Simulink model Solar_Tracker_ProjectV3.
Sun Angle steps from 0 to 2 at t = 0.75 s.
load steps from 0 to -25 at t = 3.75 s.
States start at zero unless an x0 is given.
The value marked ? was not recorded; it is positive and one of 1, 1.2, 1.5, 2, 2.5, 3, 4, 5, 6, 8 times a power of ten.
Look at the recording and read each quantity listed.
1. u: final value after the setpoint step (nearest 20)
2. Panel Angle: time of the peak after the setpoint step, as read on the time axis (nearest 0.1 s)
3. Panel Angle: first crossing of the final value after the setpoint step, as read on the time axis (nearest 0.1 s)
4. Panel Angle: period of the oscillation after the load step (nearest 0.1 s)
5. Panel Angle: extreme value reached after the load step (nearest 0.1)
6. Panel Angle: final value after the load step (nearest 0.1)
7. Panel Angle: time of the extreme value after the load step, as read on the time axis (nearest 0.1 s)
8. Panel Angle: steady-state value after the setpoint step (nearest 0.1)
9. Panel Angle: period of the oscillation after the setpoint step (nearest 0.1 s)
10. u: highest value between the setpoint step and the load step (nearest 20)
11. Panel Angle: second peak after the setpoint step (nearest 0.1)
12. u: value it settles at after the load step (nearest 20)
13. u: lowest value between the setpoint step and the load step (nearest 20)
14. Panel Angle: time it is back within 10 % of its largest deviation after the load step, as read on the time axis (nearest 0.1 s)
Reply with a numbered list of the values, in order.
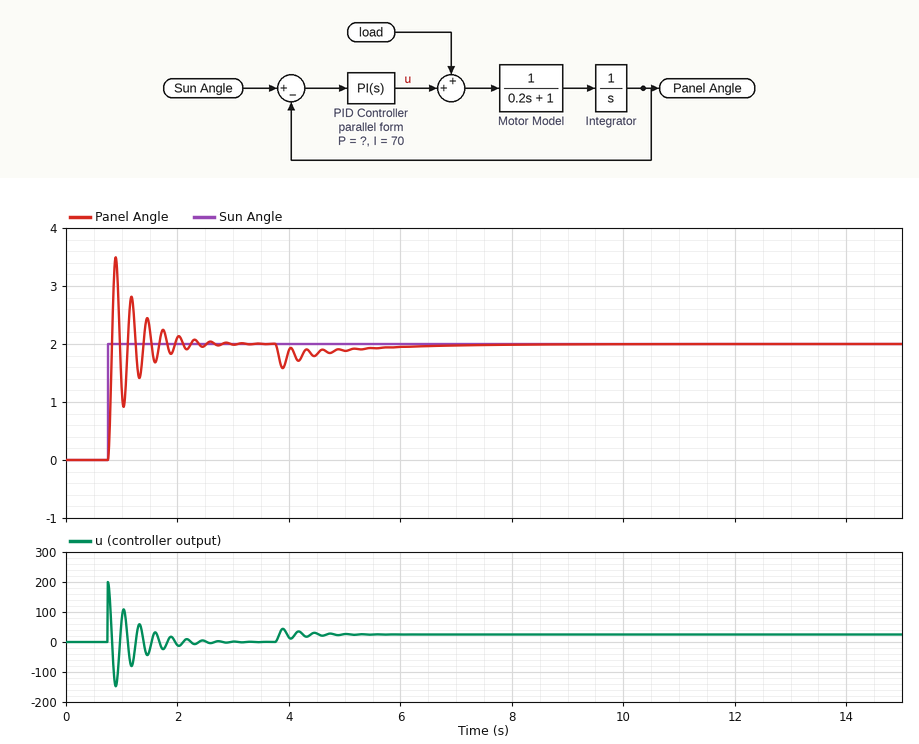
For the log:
1. 0
2. 0.9 s
3. 0.8 s
4. 0.3 s
5. 1.6
6. 2.0
7. 3.9 s
8. 2.0
9. 0.3 s
10. 200
11. 2.8
12. 20
13. -140
14. 6.3 s
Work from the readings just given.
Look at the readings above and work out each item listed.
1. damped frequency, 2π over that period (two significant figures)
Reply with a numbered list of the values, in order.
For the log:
1. 21 rad/s
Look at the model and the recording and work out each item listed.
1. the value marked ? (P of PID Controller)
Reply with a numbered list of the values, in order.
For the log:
1. 100
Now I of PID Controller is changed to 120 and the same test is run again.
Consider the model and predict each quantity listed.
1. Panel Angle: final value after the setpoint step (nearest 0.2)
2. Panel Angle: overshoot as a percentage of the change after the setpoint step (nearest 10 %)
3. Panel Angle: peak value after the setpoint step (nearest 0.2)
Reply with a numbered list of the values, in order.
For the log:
1. 2.0
2. 80 %
3. 3.6
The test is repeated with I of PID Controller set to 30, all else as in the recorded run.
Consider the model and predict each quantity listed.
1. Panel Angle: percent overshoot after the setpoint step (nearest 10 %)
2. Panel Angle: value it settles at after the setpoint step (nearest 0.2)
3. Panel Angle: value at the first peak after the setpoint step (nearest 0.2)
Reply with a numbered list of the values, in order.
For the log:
1. 70 %
2. 2.0
3. 3.4
